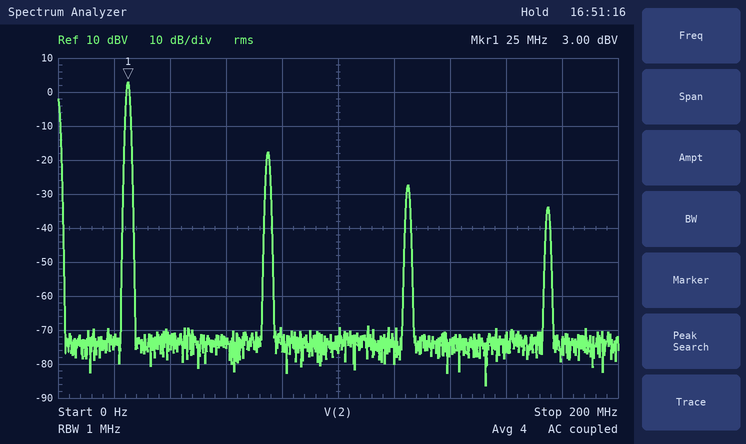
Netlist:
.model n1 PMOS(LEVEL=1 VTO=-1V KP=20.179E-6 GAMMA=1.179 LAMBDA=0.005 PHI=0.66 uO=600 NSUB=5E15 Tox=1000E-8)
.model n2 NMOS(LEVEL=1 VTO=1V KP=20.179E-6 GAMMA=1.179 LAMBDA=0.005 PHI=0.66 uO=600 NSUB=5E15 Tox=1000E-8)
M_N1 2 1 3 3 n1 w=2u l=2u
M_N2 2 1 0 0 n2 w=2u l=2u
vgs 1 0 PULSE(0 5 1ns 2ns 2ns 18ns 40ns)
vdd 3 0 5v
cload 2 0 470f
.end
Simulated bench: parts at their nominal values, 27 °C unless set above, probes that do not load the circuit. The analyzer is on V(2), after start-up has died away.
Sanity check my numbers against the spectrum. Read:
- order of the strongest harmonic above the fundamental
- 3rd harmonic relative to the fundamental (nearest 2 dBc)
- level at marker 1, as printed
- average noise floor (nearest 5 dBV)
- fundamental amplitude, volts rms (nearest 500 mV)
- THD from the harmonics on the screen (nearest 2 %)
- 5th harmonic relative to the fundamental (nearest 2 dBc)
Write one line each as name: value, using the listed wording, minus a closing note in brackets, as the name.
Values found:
order of the strongest harmonic above the fundamental: 3
3rd harmonic relative to the fundamental: -20 dBc
level at marker 1, as printed: 3.00 dBV
average noise floor: -75 dBV
fundamental amplitude, volts rms: 1.5 V
THD from the harmonics on the screen: 10 %
5th harmonic relative to the fundamental: -30 dBc
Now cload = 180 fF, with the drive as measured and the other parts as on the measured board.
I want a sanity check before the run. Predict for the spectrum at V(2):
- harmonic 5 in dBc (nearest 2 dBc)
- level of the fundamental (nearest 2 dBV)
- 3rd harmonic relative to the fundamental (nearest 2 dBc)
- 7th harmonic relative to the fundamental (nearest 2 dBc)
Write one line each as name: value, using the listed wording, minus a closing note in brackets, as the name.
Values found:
harmonic 5 in dBc: -24 dBc
level of the fundamental: 6 dBV
3rd harmonic relative to the fundamental: -14 dBc
7th harmonic relative to the fundamental: -32 dBc
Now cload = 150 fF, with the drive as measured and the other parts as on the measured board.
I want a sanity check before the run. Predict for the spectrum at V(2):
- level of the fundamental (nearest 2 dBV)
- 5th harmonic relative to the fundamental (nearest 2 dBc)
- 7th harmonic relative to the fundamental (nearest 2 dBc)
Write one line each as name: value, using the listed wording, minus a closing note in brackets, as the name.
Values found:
level of the fundamental: 6 dBV
5th harmonic relative to the fundamental: -22 dBc
7th harmonic relative to the fundamental: -30 dBc
